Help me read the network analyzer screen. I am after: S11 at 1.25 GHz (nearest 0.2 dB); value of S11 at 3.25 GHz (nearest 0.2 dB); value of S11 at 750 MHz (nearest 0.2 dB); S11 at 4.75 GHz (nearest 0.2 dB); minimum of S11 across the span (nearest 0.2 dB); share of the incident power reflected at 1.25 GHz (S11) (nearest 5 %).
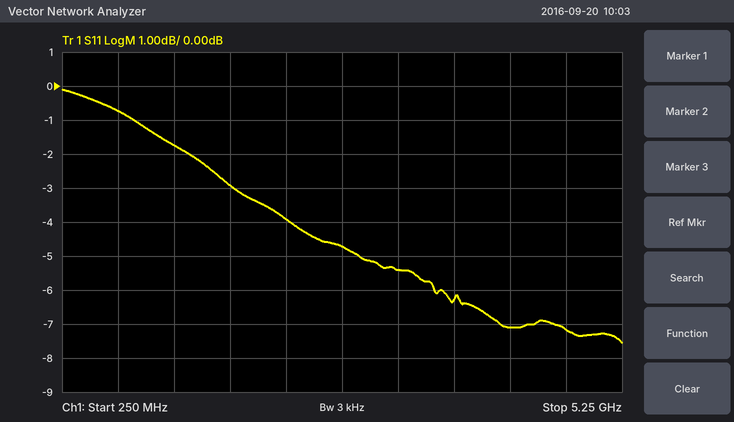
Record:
-1.8 dB
-5.4 dB
-0.8 dB
-7.2 dB
-7.6 dB
65 %
